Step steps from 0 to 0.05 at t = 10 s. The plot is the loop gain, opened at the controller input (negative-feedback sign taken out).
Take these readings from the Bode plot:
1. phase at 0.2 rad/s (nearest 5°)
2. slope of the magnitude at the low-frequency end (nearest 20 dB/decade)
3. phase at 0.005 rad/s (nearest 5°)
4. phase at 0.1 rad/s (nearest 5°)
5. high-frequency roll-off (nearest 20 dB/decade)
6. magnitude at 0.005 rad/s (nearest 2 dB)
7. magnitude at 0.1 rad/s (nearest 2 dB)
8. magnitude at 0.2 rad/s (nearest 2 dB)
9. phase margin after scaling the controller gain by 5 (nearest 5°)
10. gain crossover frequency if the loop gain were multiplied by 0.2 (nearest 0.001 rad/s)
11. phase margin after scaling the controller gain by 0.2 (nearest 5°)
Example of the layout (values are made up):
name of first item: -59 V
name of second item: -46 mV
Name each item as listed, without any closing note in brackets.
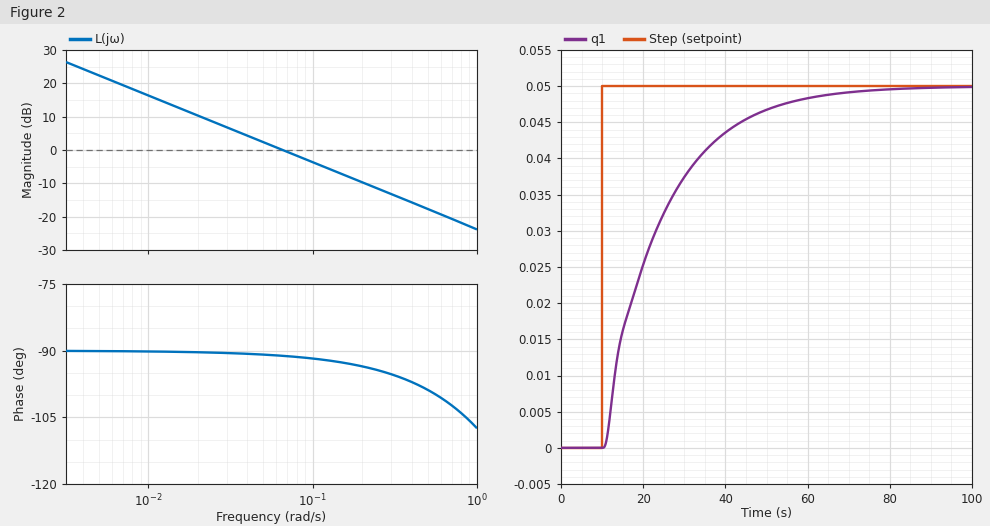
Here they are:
phase at 0.2 rad/s: -95°
slope of the magnitude at the low-frequency end: -20 dB/decade
phase at 0.005 rad/s: -90°
phase at 0.1 rad/s: -90°
high-frequency roll-off: -20 dB/decade
magnitude at 0.005 rad/s: 22 dB
magnitude at 0.1 rad/s: -4 dB
magnitude at 0.2 rad/s: -10 dB
phase margin after scaling the controller gain by 5: 85°
gain crossover frequency if the loop gain were multiplied by 0.2: 0.013 rad/s
phase margin after scaling the controller gain by 0.2: 90°
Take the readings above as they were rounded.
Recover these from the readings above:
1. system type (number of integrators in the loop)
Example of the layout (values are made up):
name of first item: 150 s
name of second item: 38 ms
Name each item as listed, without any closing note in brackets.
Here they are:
system type: 1
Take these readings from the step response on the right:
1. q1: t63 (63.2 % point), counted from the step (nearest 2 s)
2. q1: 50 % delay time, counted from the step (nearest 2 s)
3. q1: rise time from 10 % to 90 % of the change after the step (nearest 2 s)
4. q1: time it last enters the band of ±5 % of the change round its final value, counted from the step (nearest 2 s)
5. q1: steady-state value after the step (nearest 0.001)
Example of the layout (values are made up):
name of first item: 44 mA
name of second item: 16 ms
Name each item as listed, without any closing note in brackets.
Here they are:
q1: t63 (63.2 % point), counted from the step: 14 s
q1: 50 % delay time, counted from the step: 10 s
q1: rise time from 10 % to 90 % of the change after the step: 32 s
q1: time it last enters the band of ±5 % of the change round its final value, counted from the step: 44 s
q1: steady-state value after the step: 0.050
